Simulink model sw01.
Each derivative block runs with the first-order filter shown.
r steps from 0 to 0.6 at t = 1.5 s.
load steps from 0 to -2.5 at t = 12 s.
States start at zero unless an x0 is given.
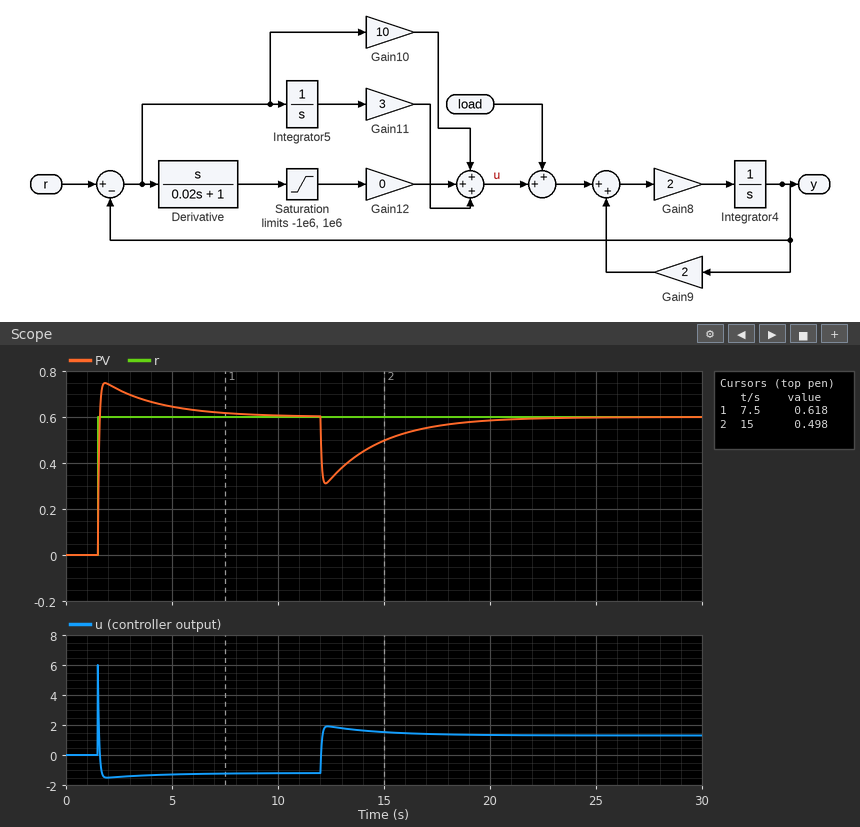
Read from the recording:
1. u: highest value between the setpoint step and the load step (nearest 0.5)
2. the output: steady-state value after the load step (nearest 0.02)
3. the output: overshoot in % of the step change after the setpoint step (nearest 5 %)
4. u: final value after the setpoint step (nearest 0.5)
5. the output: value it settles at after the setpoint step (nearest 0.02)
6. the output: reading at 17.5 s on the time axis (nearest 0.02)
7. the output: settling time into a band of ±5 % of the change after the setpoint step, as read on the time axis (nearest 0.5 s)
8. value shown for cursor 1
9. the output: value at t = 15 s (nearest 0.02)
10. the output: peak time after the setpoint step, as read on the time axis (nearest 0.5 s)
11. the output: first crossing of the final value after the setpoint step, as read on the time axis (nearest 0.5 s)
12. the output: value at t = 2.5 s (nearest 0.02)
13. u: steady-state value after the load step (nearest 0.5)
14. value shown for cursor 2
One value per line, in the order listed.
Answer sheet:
6.0
0.60
25 %
-1.0
0.60
0.56
6.0 s
0.618
0.50
2.0 s
1.5 s
0.72
1.5
0.498
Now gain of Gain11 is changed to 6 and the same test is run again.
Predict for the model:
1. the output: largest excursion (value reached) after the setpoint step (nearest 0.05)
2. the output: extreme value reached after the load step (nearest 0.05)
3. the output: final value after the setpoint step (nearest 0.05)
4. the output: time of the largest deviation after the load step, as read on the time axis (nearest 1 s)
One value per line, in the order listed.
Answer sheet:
0.75
0.30
0.60
12 s
